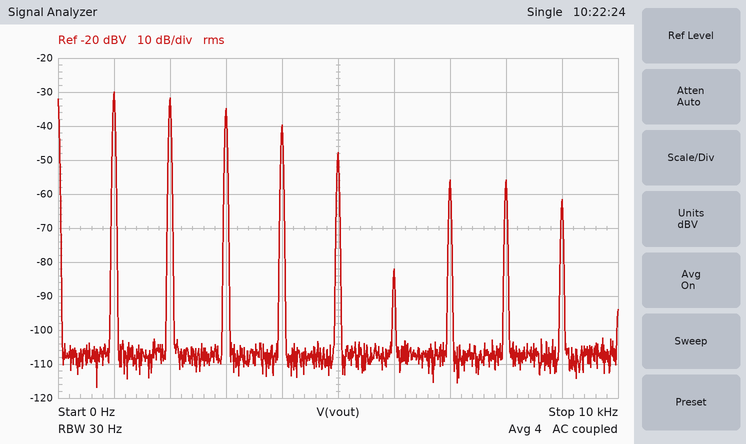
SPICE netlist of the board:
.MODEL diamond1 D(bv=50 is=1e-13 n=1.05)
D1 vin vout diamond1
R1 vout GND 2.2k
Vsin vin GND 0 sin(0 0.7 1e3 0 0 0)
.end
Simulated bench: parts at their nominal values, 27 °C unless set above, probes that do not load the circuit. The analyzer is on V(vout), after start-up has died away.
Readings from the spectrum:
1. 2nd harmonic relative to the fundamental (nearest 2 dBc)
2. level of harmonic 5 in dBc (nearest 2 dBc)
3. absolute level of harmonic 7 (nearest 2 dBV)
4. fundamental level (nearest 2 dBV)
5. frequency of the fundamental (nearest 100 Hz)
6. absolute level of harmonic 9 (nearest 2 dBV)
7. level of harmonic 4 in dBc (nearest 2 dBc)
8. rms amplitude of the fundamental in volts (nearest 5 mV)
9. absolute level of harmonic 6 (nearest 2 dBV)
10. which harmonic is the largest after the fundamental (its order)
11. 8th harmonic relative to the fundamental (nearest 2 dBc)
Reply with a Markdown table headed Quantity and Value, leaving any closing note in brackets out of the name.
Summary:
| Quantity | Value |
|---|---|
| 2nd harmonic relative to the fundamental | -2 dBc |
| level of harmonic 5 in dBc | -18 dBc |
| absolute level of harmonic 7 | -56 dBV |
| fundamental level | -30 dBV |
| frequency of the fundamental | 1.0 kHz |
| absolute level of harmonic 9 | -62 dBV |
| level of harmonic 4 in dBc | -10 dBc |
| rms amplitude of the fundamental in volts | 30 mV |
| absolute level of harmonic 6 | -82 dBV |
| which harmonic is the largest after the fundamental | 2 |
| 8th harmonic relative to the fundamental | -26 dBc |
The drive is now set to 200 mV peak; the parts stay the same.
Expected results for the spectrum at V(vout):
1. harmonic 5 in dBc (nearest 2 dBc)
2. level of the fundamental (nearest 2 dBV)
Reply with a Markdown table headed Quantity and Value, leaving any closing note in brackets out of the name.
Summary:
| Quantity | Value |
|---|---|
| harmonic 5 in dBc | -14 dBc |
| level of the fundamental | -144 dBV |
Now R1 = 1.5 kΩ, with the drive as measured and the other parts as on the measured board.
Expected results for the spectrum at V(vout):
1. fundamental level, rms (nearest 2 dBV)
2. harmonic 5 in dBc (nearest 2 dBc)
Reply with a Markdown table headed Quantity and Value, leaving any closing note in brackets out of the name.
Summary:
| Quantity | Value |
|---|---|
| fundamental level, rms | -30 dBV |
| harmonic 5 in dBc | -16 dBc |
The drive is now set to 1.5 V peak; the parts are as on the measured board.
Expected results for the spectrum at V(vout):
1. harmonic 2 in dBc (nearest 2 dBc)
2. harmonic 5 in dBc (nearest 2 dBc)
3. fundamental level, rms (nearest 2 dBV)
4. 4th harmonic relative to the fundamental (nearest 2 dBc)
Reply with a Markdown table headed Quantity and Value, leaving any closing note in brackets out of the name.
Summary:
| Quantity | Value |
|---|---|
| harmonic 2 in dBc | -4 dBc |
| harmonic 5 in dBc | -22 dBc |
| fundamental level, rms | -12 dBV |
| 4th harmonic relative to the fundamental | -34 dBc |
